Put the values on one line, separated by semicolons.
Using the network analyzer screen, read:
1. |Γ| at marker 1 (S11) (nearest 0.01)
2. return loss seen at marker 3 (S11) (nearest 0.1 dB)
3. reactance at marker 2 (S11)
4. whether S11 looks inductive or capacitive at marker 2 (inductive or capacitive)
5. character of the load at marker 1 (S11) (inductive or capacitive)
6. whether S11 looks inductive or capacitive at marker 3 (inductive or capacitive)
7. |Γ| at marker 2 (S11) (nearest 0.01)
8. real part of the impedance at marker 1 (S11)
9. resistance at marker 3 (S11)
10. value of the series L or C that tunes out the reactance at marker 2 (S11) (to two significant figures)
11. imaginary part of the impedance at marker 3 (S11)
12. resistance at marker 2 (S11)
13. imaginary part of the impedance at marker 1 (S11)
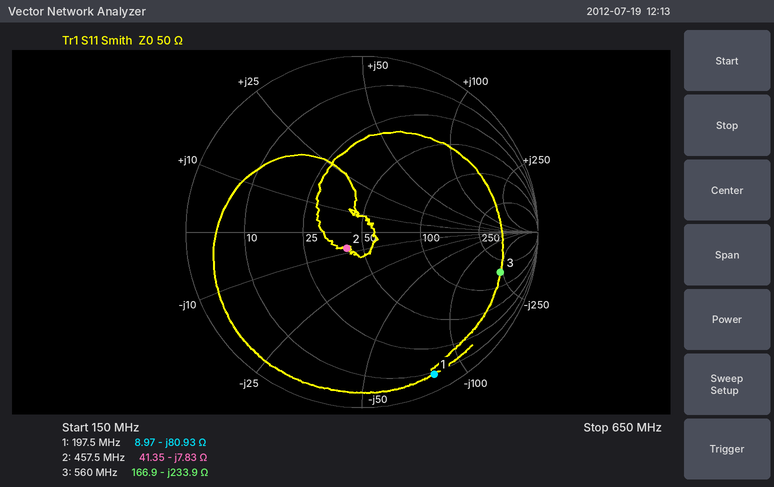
0.91; 1.7 dB; -7.83 Ω; capacitive; capacitive; capacitive; 0.13; 8.97 Ω; 166.9 Ω; 2.7 nH; -233.9 Ω; 41.35 Ω; -80.93 Ω
